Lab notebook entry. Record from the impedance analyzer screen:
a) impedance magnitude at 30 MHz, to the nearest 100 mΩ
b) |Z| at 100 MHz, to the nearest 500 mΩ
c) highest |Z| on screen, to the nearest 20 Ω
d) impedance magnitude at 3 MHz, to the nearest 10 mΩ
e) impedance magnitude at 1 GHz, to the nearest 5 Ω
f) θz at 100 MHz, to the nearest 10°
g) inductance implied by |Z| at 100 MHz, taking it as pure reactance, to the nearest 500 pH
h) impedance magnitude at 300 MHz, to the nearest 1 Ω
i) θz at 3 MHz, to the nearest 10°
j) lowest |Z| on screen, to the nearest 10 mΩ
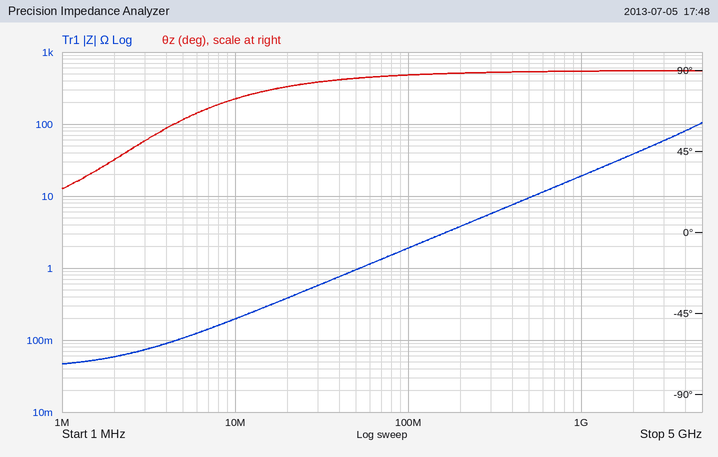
600 mΩ
2.0 Ω
100 Ω
70 mΩ
20 Ω
90°
3.0 nH
6 Ω
50°
50 mΩ
